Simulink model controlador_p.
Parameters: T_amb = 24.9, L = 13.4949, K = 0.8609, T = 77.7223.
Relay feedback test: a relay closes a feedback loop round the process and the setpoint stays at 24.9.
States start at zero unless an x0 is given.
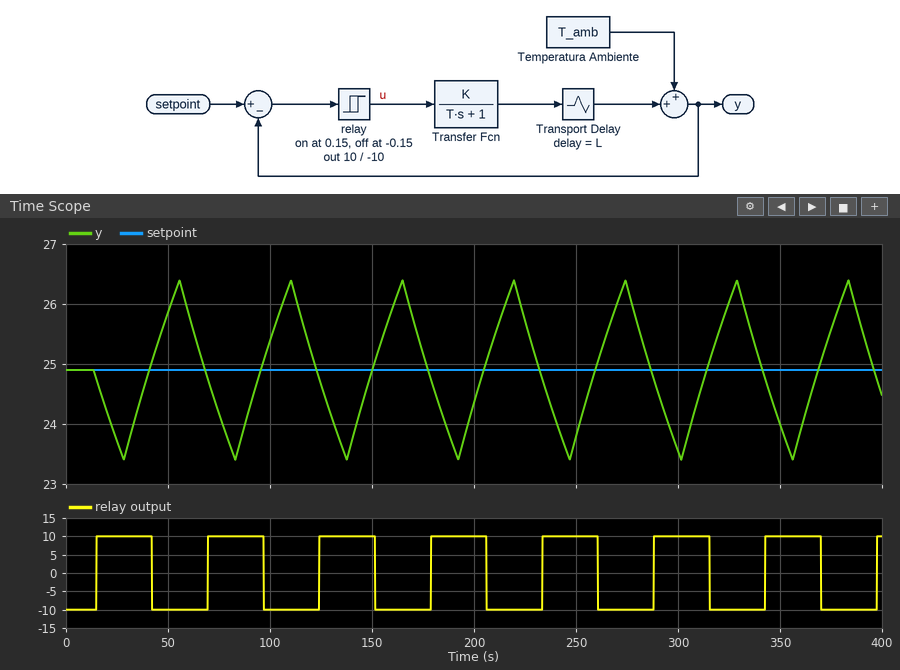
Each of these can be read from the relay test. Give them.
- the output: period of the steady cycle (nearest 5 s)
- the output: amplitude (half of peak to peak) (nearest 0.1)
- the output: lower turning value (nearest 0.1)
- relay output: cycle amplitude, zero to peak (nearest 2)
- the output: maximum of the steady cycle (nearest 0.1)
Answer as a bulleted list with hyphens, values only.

- 55 s
- 1.5
- 23.4
- 10
- 26.4
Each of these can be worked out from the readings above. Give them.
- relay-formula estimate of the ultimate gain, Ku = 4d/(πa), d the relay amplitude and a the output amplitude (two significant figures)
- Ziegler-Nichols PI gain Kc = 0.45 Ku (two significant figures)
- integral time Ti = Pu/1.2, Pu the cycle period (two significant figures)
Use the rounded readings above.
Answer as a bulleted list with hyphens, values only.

- 8.5
- 3.8
- 46 s
